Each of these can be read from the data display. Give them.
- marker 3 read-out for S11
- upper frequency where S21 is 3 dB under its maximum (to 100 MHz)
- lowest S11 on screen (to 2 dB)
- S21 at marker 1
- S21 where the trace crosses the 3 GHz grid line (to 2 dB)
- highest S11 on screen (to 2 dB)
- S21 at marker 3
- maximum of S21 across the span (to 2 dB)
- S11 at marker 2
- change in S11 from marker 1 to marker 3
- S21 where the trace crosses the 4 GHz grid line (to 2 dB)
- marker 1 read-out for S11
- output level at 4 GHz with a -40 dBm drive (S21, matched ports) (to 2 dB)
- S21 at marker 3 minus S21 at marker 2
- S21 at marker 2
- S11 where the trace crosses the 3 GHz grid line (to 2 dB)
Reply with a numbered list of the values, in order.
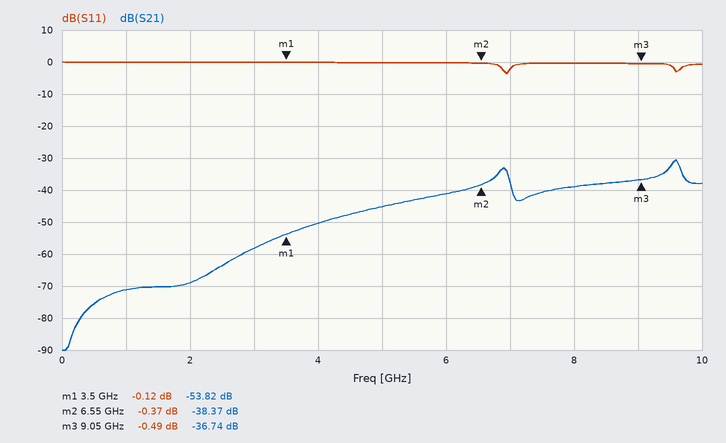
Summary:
1. -0.49 dB
2. 9.7 GHz
3. -4 dB
4. -53.82 dB
5. -58 dB
6. 0 dB
7. -36.74 dB
8. -30 dB
9. -0.37 dB
10. -0.37 dB
11. -50 dB
12. -0.12 dB
13. -90 dBm
14. 1.63 dB
15. -38.37 dB
16. 0 dB
